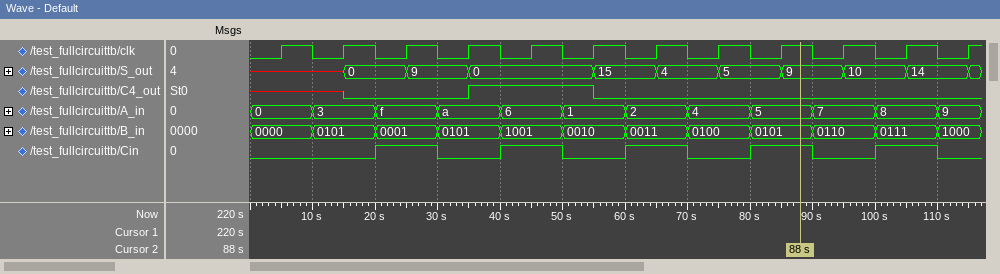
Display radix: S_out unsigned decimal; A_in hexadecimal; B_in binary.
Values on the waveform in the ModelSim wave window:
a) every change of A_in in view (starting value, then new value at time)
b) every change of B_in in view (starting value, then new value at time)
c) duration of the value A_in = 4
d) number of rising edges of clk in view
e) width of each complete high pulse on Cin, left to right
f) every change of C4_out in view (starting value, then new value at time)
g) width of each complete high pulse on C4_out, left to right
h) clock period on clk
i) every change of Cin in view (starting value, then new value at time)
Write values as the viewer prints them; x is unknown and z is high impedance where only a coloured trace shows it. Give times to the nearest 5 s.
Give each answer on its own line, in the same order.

0, 3 at 10 s, f at 20 s, a at 30 s, 6 at 40 s, 1 at 50 s, 2 at 60 s, 4 at 70 s, 5 at 80 s, 7 at 90 s, 8 at 100 s, 9 at 110 s
0000, 0101 at 10 s, 0001 at 20 s, 0101 at 30 s, 1001 at 40 s, 0010 at 50 s, 0011 at 60 s, 0100 at 70 s, 0101 at 80 s, 0110 at 90 s, 0111 at 100 s, 1000 at 110 s
10 s
12
10 s, 10 s, 10 s, 10 s, 10 s
x, 0 at 15 s, 1 at 35 s, 0 at 55 s
20 s
10 s
0, 1 at 20 s, 0 at 30 s, 1 at 40 s, 0 at 50 s, 1 at 60 s, 0 at 70 s, 1 at 80 s, 0 at 90 s, 1 at 100 s, 0 at 110 s
